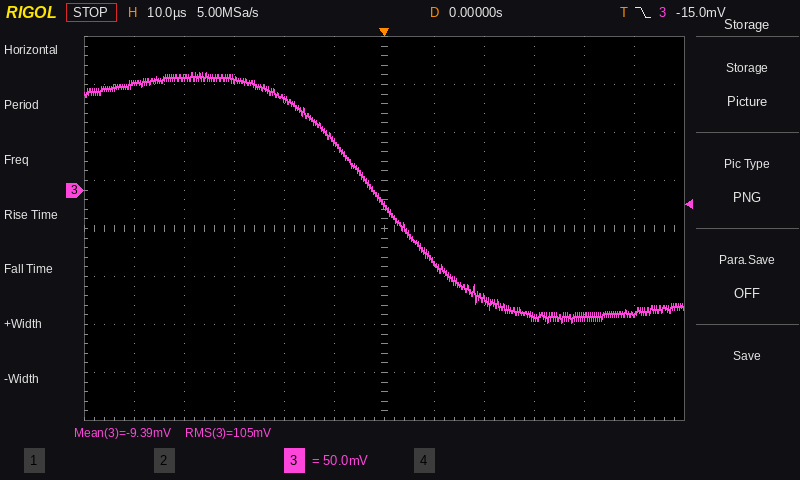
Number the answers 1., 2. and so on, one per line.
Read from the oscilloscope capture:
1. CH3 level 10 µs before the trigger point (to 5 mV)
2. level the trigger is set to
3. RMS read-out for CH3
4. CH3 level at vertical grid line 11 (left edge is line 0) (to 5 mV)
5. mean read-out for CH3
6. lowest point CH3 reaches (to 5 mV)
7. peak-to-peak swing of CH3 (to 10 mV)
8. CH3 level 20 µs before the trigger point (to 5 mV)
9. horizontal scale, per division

1. 50 mV
2. -15.0 mV
3. 105 mV
4. -130 mV
5. -9.39 mV
6. -140 mV
7. 260 mV
8. 95 mV
9. 10 µs
